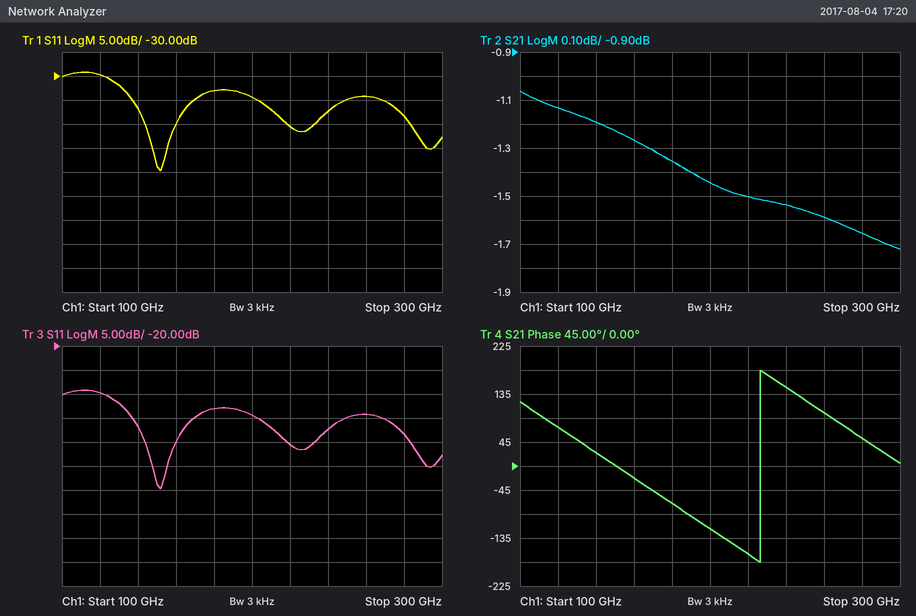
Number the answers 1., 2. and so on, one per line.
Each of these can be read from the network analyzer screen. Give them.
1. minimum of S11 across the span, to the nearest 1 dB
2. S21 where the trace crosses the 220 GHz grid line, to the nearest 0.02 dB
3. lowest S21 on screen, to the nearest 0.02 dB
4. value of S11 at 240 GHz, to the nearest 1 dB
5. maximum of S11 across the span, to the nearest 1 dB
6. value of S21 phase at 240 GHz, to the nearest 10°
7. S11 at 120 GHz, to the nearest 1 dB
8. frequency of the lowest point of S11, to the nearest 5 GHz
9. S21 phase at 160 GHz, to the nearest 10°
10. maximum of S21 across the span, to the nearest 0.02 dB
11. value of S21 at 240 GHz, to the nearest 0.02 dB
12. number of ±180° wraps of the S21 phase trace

1. -50 dB
2. -1.50 dB
3. -1.72 dB
4. -37 dB
5. -29 dB
6. 150°
7. -30 dB
8. 150 GHz
9. -20°
10. -1.06 dB
11. -1.54 dB
12. 1
